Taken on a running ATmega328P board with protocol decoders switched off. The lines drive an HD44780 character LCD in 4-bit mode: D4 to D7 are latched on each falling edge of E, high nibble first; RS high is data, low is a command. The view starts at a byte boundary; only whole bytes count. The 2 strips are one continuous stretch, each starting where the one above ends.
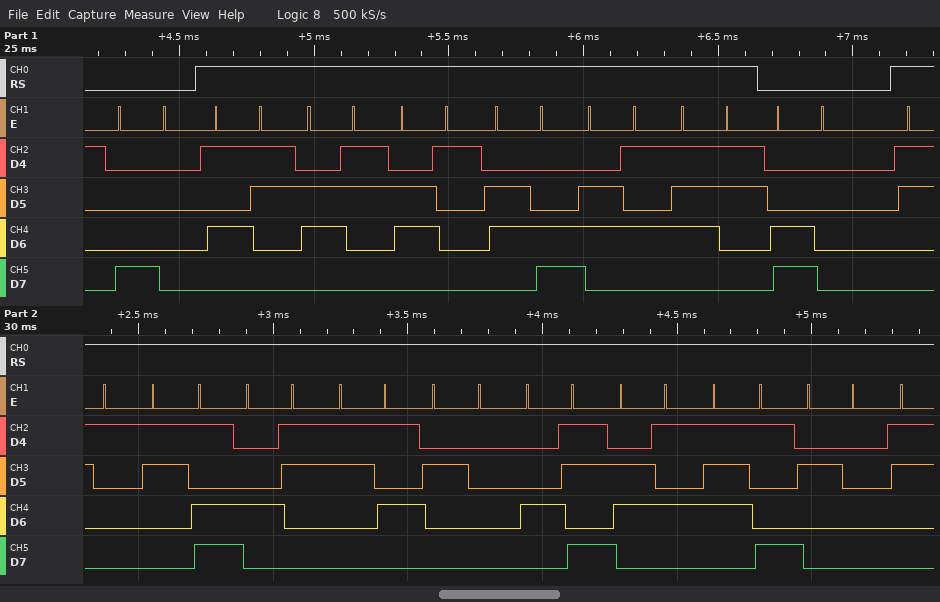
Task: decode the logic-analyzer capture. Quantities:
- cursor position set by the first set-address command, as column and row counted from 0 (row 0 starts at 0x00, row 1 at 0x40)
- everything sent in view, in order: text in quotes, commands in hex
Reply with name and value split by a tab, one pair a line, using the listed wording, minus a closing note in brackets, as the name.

cursor position set by the first set-address command, as column and row counted from 0	column 0, row 0
everything sent in view, in order: text in quotes, commands in hex	0x80 "Scales" 0xC0 "1=C5 Key "
